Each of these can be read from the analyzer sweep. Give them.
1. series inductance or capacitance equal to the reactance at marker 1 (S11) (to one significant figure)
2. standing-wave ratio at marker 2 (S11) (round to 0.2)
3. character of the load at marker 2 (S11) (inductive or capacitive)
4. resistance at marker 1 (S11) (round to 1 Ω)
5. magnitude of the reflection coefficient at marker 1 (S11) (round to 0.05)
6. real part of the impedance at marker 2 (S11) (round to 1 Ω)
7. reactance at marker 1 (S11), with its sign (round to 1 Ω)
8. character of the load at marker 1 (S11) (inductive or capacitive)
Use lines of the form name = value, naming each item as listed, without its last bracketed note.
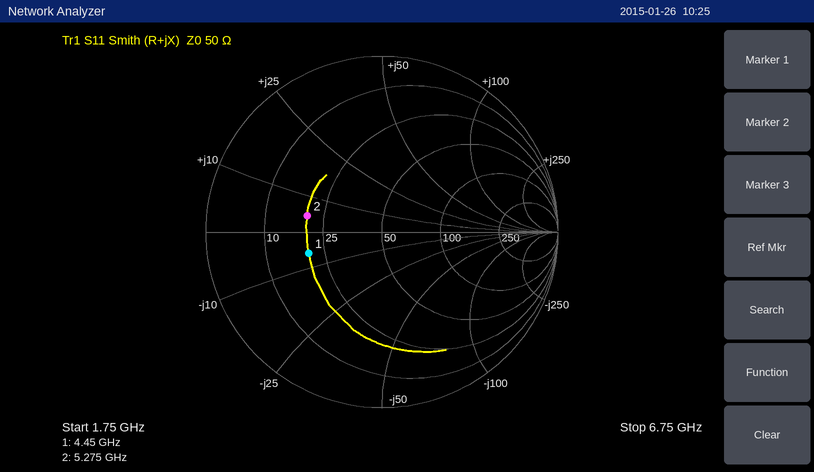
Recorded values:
series inductance or capacitance equal to the reactance at marker 1 (S11) = 6 pF
standing-wave ratio at marker 2 (S11) = 2.6
character of the load at marker 2 (S11) = inductive
resistance at marker 1 (S11) = 20 Ω
magnitude of the reflection coefficient at marker 1 (S11) = 0.45
real part of the impedance at marker 2 (S11) = 20 Ω
reactance at marker 1 (S11), with its sign = -6 Ω
character of the load at marker 1 (S11) = capacitive
